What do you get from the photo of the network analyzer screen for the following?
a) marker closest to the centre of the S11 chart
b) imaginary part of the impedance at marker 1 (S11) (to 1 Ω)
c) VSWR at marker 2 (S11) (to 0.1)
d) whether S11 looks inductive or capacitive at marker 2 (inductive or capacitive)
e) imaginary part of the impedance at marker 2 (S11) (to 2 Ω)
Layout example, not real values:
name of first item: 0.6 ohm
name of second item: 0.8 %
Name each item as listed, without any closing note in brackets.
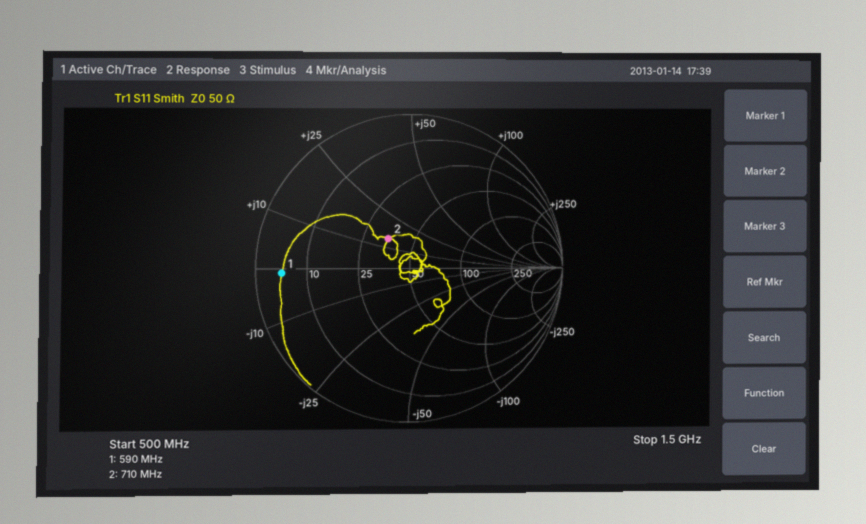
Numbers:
marker closest to the centre of the S11 chart: marker 2
imaginary part of the impedance at marker 1 (S11): -1 Ω
VSWR at marker 2 (S11): 1.6
whether S11 looks inductive or capacitive at marker 2: inductive
imaginary part of the impedance at marker 2 (S11): +14 Ω
